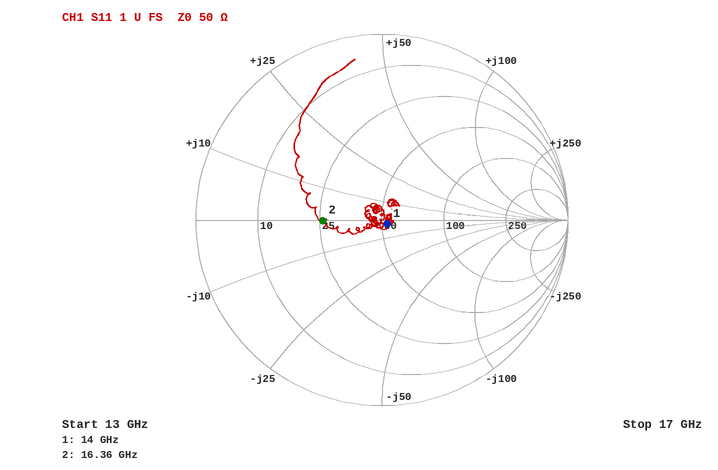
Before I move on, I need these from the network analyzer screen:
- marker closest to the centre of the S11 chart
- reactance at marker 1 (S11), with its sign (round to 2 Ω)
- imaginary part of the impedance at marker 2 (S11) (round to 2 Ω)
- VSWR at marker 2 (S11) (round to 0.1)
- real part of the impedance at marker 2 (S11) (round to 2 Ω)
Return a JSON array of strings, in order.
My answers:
["marker 1", "-2 Ω", "0 Ω", "1.9", "26 Ω"]
